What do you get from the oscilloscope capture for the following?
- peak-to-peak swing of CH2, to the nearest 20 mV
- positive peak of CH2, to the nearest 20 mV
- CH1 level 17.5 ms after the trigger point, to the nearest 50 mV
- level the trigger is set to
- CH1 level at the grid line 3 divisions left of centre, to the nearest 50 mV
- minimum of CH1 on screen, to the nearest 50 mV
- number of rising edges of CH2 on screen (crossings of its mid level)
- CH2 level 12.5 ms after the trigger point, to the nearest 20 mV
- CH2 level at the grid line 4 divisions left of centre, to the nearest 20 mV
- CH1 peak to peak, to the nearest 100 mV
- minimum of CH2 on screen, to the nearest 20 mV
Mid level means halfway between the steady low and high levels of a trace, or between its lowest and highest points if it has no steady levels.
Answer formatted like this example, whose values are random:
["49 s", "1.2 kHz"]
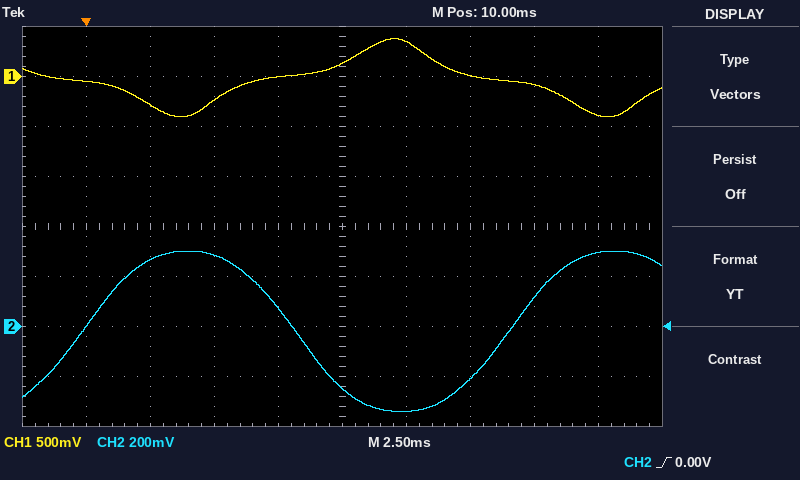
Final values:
["640 mV", "300 mV", "-100 mV", "0.00 V", "-300 mV", "-400 mV", "2", "-340 mV", "0 mV", "800 mV", "-340 mV"]
